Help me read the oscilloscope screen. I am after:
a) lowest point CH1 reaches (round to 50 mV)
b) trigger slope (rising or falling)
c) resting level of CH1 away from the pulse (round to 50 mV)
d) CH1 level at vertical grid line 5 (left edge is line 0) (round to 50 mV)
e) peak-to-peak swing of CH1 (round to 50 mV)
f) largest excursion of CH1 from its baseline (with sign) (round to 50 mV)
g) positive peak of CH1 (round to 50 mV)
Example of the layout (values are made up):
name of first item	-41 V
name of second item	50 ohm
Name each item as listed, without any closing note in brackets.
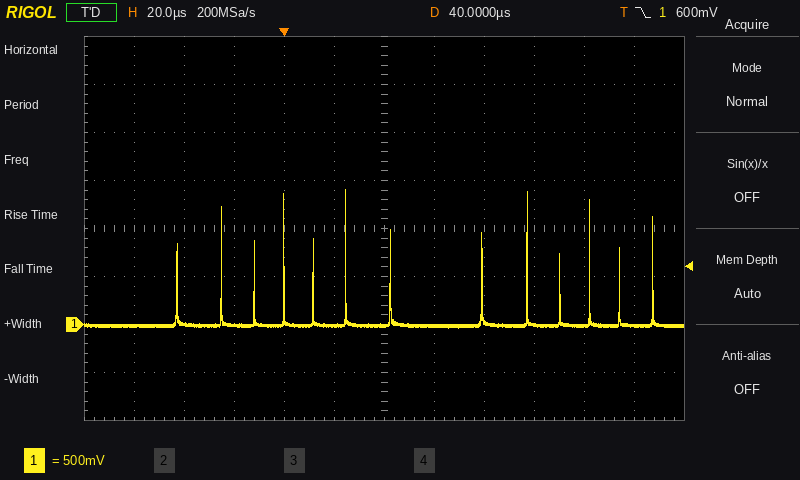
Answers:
lowest point CH1 reaches	-50 mV
trigger slope	falling
resting level of CH1 away from the pulse	0 mV
CH1 level at vertical grid line 5 (left edge is line 0)	0 mV
peak-to-peak swing of CH1	1.45 V
largest excursion of CH1 from its baseline (with sign)	+1.40 V
positive peak of CH1	1.40 V
